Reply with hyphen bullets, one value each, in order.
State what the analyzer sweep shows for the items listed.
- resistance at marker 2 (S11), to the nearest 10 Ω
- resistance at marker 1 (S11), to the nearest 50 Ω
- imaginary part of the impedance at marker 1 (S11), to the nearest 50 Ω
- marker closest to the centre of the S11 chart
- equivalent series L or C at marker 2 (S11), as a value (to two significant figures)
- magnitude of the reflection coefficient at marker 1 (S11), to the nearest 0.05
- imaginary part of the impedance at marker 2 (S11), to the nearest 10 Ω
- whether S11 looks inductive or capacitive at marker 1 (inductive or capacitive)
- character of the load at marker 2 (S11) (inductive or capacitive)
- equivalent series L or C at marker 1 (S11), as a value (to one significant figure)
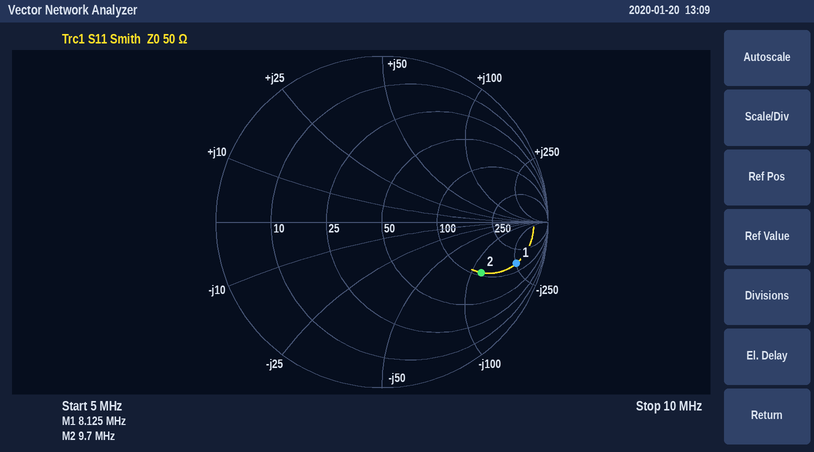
- 110 Ω
- 150 Ω
- -250 Ω
- marker 2
- 140 pF
- 0.85
- -120 Ω
- capacitive
- capacitive
- 80 pF
